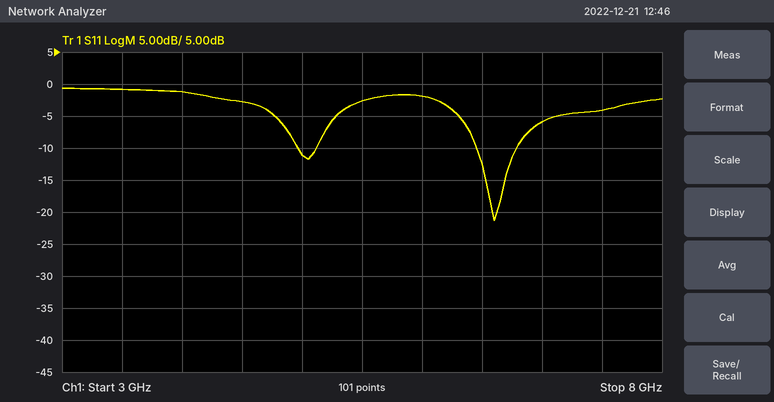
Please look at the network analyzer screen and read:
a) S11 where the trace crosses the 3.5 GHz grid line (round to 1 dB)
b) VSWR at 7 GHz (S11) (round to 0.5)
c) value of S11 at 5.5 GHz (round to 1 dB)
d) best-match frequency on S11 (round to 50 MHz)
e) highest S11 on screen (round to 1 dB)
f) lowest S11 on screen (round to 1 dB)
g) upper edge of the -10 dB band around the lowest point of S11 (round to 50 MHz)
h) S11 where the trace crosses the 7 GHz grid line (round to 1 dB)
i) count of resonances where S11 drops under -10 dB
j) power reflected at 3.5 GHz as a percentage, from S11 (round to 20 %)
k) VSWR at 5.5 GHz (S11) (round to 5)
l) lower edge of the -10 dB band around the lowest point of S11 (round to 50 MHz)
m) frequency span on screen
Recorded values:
-1 dB
3.0
-3 dB
6.60 GHz
-1 dB
-21 dB
6.80 GHz
-6 dB
2
80 %
5
6.45 GHz
5 GHz
